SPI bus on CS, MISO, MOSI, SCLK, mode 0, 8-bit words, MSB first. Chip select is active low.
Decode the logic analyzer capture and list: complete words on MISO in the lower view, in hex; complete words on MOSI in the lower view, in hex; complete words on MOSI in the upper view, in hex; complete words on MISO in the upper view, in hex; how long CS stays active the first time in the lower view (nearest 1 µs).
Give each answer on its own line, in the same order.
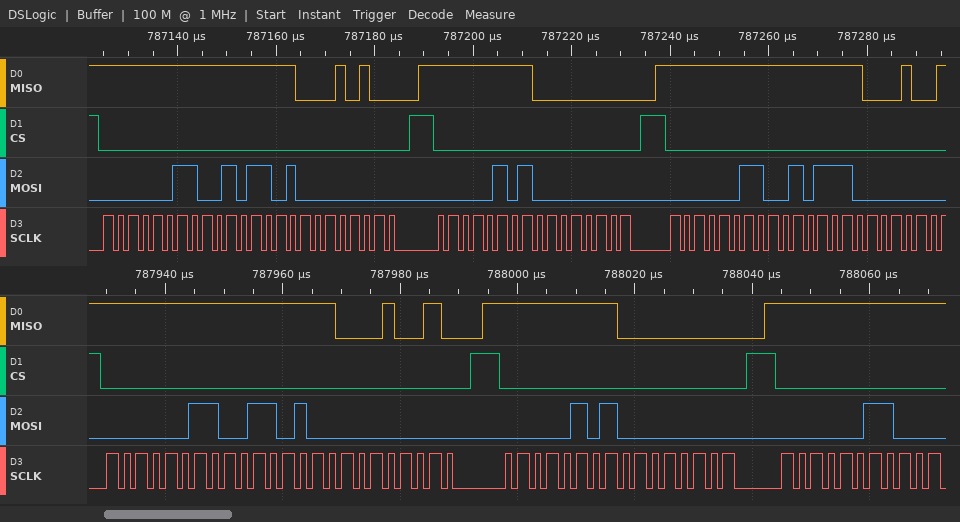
FF, FF, 12, FF, 00, FF
03, 34, 00, 05, 00, 03
03, 2D, 00, 05, 00, 03, 2E
FF, FF, 14, FF, 00, FF, FF
63 µs
